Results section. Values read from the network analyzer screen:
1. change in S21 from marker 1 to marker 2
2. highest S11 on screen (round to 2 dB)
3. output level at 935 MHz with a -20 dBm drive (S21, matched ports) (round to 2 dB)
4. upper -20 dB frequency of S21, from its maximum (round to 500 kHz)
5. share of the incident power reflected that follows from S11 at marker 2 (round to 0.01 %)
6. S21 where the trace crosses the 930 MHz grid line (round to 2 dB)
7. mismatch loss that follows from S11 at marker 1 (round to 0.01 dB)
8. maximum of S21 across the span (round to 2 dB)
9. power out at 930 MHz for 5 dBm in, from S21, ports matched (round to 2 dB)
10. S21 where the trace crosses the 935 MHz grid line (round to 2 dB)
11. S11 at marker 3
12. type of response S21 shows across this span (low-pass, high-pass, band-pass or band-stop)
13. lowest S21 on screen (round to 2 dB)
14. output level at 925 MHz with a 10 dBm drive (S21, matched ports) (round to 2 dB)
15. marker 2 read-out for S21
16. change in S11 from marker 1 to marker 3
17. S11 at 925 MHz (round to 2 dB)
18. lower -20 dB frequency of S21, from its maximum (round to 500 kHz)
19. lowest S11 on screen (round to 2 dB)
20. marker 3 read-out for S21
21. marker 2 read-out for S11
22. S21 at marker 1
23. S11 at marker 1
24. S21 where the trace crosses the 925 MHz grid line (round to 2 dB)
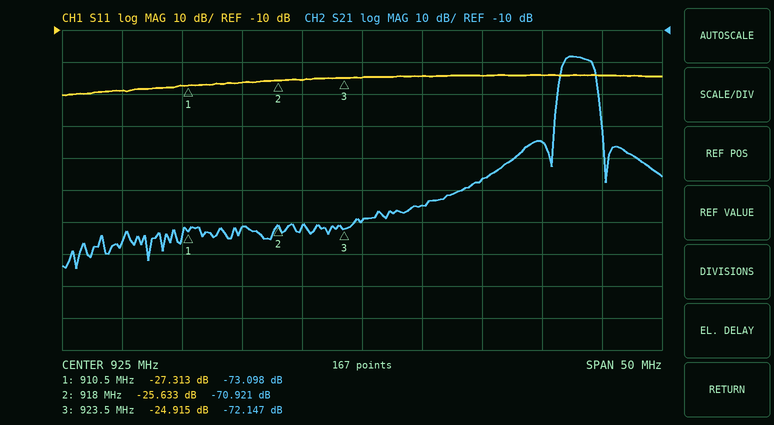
2.177 dB
-24 dB
-76 dBm
945.0 MHz
0.27 %
-64 dB
0.01 dB
-18 dB
-60 dBm
-56 dB
-24.915 dB
band-pass
-84 dB
-60 dBm
-70.921 dB
2.398 dB
-24 dB
941.0 MHz
-30 dB
-72.147 dB
-25.633 dB
-73.098 dB
-27.313 dB
-70 dB
